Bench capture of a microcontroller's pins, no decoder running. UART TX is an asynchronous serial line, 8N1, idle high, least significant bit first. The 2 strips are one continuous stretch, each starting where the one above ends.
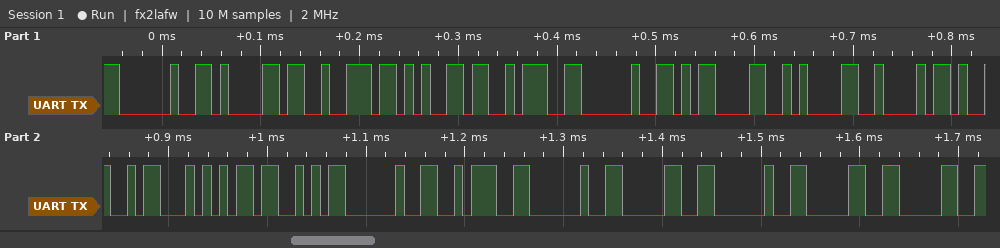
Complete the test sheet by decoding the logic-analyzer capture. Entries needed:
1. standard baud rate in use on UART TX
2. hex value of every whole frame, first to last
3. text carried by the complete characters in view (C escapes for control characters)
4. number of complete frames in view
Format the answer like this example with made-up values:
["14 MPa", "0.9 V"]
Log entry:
["115200 baud", "20 61 72 65 3A 20 0D 0A 42 49 54 53 20 3A 20 30 20 30 30", "\" are: \\r\\nBITS : 0 00\"", "19"]
